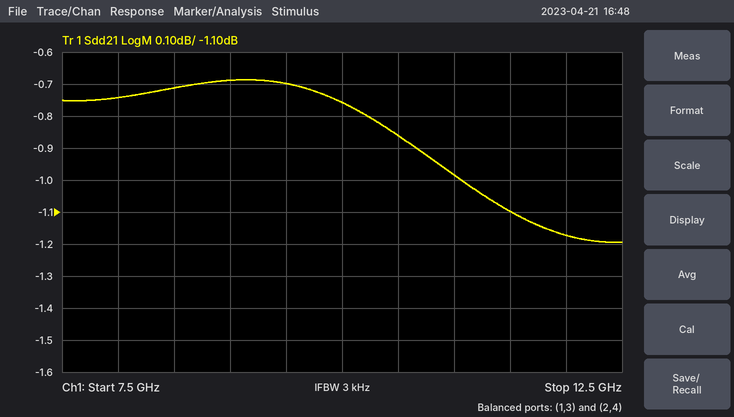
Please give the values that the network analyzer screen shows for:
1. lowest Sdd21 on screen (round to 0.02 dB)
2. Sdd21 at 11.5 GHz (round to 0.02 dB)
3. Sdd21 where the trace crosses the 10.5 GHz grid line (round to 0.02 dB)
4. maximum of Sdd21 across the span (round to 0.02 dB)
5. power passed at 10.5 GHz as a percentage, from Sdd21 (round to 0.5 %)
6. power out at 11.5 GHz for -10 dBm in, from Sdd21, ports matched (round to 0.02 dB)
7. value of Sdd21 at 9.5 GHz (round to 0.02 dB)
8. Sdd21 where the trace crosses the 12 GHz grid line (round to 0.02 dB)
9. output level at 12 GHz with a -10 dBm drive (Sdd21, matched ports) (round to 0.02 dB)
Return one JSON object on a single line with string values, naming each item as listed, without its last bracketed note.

{"lowest Sdd21 on screen": "-1.20 dB", "Sdd21 at 11.5 GHz": "-1.10 dB", "Sdd21 where the trace crosses the 10.5 GHz grid line": "-0.86 dB", "maximum of Sdd21 across the span": "-0.68 dB", "power passed at 10.5 GHz as a percentage, from Sdd21": "82.0 %", "power out at 11.5 GHz for -10 dBm in, from Sdd21, ports matched": "-11.10 dBm", "value of Sdd21 at 9.5 GHz": "-0.70 dB", "Sdd21 where the trace crosses the 12 GHz grid line": "-1.18 dB", "output level at 12 GHz with a -10 dBm drive (Sdd21, matched ports)": "-11.18 dBm"}
